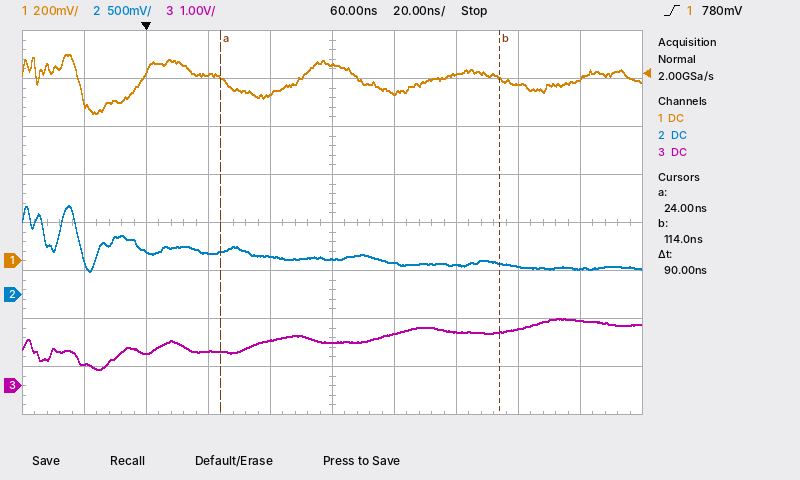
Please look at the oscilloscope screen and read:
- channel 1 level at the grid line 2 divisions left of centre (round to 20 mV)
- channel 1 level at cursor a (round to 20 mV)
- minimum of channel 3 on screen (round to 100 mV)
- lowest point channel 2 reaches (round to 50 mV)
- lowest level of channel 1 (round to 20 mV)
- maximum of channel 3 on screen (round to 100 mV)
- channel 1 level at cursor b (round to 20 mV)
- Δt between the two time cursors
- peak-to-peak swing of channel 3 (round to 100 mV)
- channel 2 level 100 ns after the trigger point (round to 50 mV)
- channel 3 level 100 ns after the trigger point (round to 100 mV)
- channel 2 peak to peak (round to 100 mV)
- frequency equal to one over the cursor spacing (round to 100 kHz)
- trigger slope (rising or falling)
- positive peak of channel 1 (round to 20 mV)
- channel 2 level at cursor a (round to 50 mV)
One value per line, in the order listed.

780 mV
760 mV
300 mV
250 mV
620 mV
1.4 V
760 mV
90 ns
1.1 V
300 mV
1.1 V
700 mV
11.1 MHz
rising
860 mV
450 mV
